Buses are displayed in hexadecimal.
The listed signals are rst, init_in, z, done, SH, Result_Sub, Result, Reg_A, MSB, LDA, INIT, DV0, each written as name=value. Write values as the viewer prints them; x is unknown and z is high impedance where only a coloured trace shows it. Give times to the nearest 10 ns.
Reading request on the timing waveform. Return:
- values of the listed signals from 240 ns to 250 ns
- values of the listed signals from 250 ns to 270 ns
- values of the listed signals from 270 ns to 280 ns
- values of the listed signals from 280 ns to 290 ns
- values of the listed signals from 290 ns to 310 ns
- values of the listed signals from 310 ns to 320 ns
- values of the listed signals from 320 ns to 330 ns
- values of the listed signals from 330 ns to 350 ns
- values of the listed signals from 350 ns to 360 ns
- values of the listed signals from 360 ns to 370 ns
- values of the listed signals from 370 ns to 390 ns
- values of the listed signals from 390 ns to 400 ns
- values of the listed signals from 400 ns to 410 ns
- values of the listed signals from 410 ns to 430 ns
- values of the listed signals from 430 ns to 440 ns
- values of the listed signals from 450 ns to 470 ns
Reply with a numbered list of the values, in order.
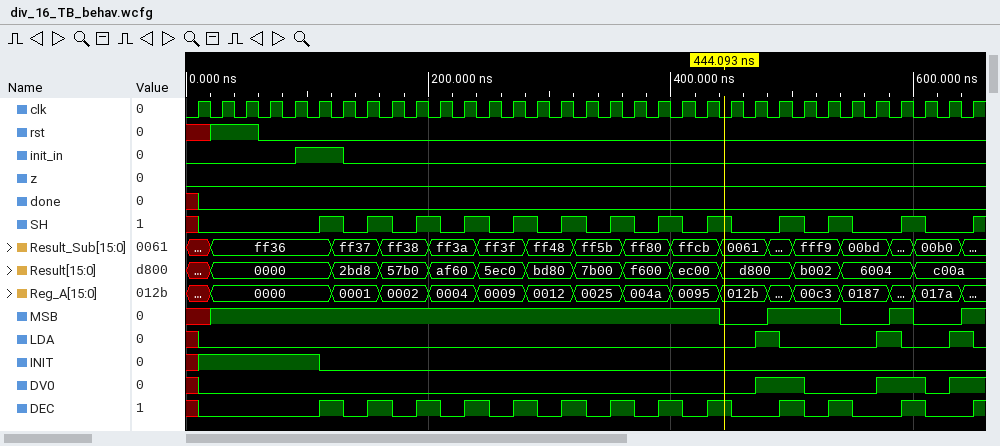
1. rst=0, init_in=0, z=0, done=0, SH=1, Result_Sub=ff3f, Result=5ec0, Reg_A=0009, MSB=1, LDA=0, INIT=0, DV0=0
2. rst=0, init_in=0, z=0, done=0, SH=0, Result_Sub=ff3f, Result=5ec0, Reg_A=0009, MSB=1, LDA=0, INIT=0, DV0=0
3. rst=0, init_in=0, z=0, done=0, SH=1, Result_Sub=ff3f, Result=5ec0, Reg_A=0009, MSB=1, LDA=0, INIT=0, DV0=0
4. rst=0, init_in=0, z=0, done=0, SH=1, Result_Sub=ff48, Result=bd80, Reg_A=0012, MSB=1, LDA=0, INIT=0, DV0=0
5. rst=0, init_in=0, z=0, done=0, SH=0, Result_Sub=ff48, Result=bd80, Reg_A=0012, MSB=1, LDA=0, INIT=0, DV0=0
6. rst=0, init_in=0, z=0, done=0, SH=1, Result_Sub=ff48, Result=bd80, Reg_A=0012, MSB=1, LDA=0, INIT=0, DV0=0
7. rst=0, init_in=0, z=0, done=0, SH=1, Result_Sub=ff5b, Result=7b00, Reg_A=0025, MSB=1, LDA=0, INIT=0, DV0=0
8. rst=0, init_in=0, z=0, done=0, SH=0, Result_Sub=ff5b, Result=7b00, Reg_A=0025, MSB=1, LDA=0, INIT=0, DV0=0
9. rst=0, init_in=0, z=0, done=0, SH=1, Result_Sub=ff5b, Result=7b00, Reg_A=0025, MSB=1, LDA=0, INIT=0, DV0=0
10. rst=0, init_in=0, z=0, done=0, SH=1, Result_Sub=ff80, Result=f600, Reg_A=004a, MSB=1, LDA=0, INIT=0, DV0=0
11. rst=0, init_in=0, z=0, done=0, SH=0, Result_Sub=ff80, Result=f600, Reg_A=004a, MSB=1, LDA=0, INIT=0, DV0=0
12. rst=0, init_in=0, z=0, done=0, SH=1, Result_Sub=ff80, Result=f600, Reg_A=004a, MSB=1, LDA=0, INIT=0, DV0=0
13. rst=0, init_in=0, z=0, done=0, SH=1, Result_Sub=ffcb, Result=ec00, Reg_A=0095, MSB=1, LDA=0, INIT=0, DV0=0
14. rst=0, init_in=0, z=0, done=0, SH=0, Result_Sub=ffcb, Result=ec00, Reg_A=0095, MSB=1, LDA=0, INIT=0, DV0=0
15. rst=0, init_in=0, z=0, done=0, SH=1, Result_Sub=ffcb, Result=ec00, Reg_A=0095, MSB=1, LDA=0, INIT=0, DV0=0
16. rst=0, init_in=0, z=0, done=0, SH=0, Result_Sub=0061, Result=d800, Reg_A=012b, MSB=0, LDA=0, INIT=0, DV0=0
